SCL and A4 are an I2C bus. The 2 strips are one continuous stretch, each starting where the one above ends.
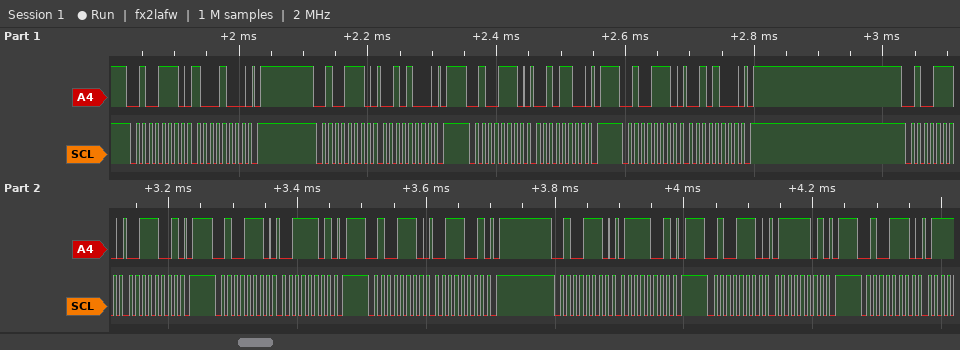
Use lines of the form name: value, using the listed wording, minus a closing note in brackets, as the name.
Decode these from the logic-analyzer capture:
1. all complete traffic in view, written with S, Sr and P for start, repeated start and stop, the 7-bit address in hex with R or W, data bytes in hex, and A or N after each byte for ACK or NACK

all complete traffic in view, written with S, Sr and P for start, repeated start and stop, the 7-bit address in hex with R or W, data bytes in hex, and A or N after each byte for ACK or NACK: S 27W A 88 A P S 27W A 28 A P S 27W A 2C A P S 27W A 28 A P S 27W A 39 A P S 27W A 3D A P S 27W A 39 A P S 27W A 79 A P S 27W A 7D A P S 27W A
